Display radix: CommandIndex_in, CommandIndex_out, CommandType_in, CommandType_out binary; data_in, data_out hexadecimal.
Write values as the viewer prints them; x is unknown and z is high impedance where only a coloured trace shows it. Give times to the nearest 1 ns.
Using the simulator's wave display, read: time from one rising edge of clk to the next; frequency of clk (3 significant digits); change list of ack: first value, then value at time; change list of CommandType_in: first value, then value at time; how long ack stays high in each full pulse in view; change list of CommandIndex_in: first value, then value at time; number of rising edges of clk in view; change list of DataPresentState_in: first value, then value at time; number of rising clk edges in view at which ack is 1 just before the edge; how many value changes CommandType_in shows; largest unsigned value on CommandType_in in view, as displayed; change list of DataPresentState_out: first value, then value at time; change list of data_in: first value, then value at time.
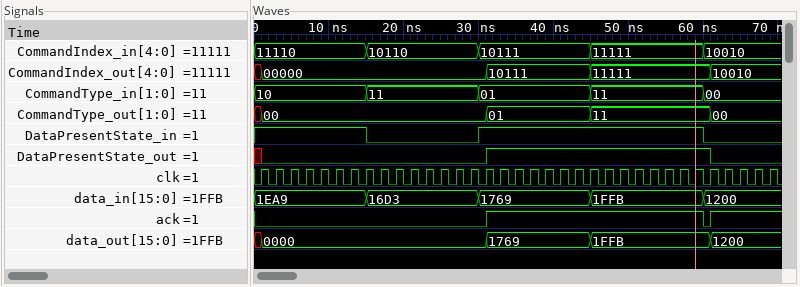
2 ns
500 MHz
0, 1 at 31 ns, 0 at 60 ns, 1 at 61 ns
10, 11 at 15 ns, 01 at 30 ns, 11 at 45 ns, 00 at 60 ns
29 ns
11110, 10110 at 15 ns, 10111 at 30 ns, 11111 at 45 ns, 10010 at 60 ns
35
1, 0 at 15 ns, 1 at 30 ns, 0 at 60 ns
18
4
11
x, 0 at 1 ns, 1 at 31 ns, 0 at 61 ns
1EA9, 16D3 at 15 ns, 1769 at 30 ns, 1FFB at 45 ns, 1200 at 60 ns
